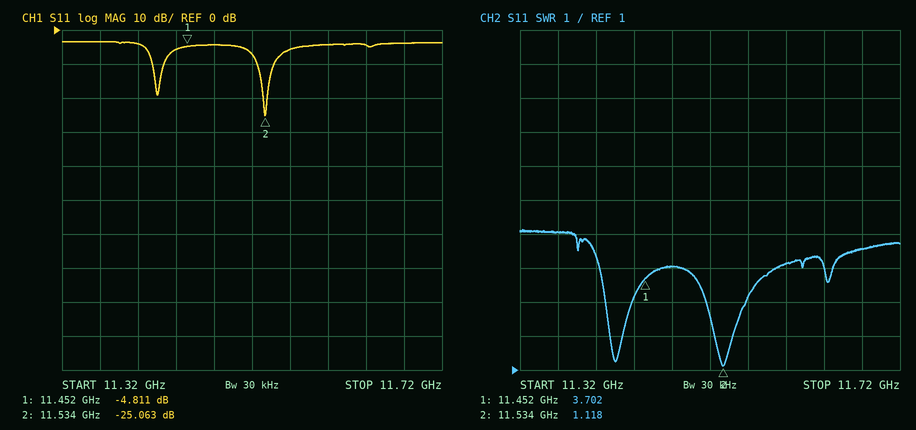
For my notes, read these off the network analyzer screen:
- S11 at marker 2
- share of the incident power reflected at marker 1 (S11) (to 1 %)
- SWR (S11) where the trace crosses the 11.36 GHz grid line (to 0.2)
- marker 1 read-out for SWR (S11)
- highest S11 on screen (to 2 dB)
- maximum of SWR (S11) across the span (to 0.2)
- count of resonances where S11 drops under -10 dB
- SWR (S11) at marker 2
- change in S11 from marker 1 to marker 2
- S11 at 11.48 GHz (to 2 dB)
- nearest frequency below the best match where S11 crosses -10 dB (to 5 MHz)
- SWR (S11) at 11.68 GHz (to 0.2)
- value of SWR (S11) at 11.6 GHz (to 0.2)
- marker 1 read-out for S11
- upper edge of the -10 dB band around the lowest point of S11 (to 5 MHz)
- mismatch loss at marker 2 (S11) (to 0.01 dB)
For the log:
-25.063 dB
33 %
5.0
3.702
-4 dB
5.2
2
1.118
-20.252 dB
-4 dB
11.525 GHz
4.6
4.2
-4.811 dB
11.545 GHz
0.01 dB
